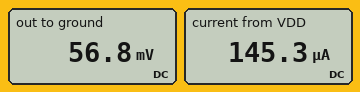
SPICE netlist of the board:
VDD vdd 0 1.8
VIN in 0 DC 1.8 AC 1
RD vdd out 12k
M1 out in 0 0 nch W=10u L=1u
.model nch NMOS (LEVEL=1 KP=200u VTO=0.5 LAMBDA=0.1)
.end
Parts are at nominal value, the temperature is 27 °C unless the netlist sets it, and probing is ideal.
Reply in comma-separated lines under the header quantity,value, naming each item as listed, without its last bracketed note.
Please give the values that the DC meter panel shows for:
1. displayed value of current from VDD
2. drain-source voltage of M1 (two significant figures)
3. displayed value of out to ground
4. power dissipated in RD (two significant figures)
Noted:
quantity,value
displayed value of current from VDD,145.3 µA
drain-source voltage of M1,57 mV
displayed value of out to ground,56.8 mV
power dissipated in RD,250 µW
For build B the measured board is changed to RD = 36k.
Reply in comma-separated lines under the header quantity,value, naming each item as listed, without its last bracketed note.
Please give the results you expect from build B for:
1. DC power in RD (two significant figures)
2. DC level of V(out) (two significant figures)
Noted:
quantity,value
DC power in RD,88 µW
DC level of V(out),19 mV
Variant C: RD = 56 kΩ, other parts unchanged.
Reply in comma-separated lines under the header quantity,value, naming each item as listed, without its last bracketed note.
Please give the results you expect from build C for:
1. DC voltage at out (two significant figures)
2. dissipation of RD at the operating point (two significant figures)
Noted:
quantity,value
DC voltage at out,12 mV
dissipation of RD at the operating point,57 µW
